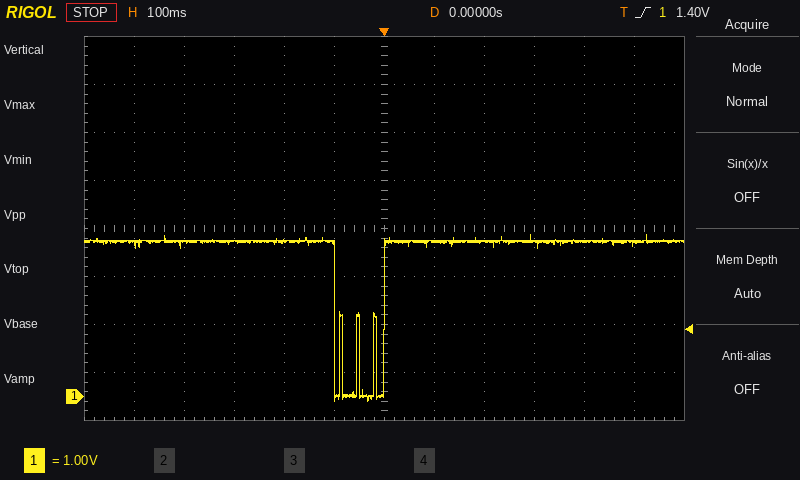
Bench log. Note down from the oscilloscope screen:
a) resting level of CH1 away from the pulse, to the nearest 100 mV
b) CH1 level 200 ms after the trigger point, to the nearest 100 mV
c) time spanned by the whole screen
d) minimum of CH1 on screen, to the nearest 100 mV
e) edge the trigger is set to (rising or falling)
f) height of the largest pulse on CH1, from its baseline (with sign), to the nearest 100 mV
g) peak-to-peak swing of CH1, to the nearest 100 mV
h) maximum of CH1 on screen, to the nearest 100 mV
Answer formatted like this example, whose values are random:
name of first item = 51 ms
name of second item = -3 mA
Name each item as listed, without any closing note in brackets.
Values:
resting level of CH1 away from the pulse, to the nearest 100 mV = 3.2 V
CH1 level 200 ms after the trigger point, to the nearest 100 mV = 3.2 V
time spanned by the whole screen = 1.2 s
minimum of CH1 on screen, to the nearest 100 mV = -100 mV
edge the trigger is set to = rising
height of the largest pulse on CH1, from its baseline (with sign), to the nearest 100 mV = -3.3 V
peak-to-peak swing of CH1, to the nearest 100 mV = 3.5 V
maximum of CH1 on screen, to the nearest 100 mV = 3.4 V
